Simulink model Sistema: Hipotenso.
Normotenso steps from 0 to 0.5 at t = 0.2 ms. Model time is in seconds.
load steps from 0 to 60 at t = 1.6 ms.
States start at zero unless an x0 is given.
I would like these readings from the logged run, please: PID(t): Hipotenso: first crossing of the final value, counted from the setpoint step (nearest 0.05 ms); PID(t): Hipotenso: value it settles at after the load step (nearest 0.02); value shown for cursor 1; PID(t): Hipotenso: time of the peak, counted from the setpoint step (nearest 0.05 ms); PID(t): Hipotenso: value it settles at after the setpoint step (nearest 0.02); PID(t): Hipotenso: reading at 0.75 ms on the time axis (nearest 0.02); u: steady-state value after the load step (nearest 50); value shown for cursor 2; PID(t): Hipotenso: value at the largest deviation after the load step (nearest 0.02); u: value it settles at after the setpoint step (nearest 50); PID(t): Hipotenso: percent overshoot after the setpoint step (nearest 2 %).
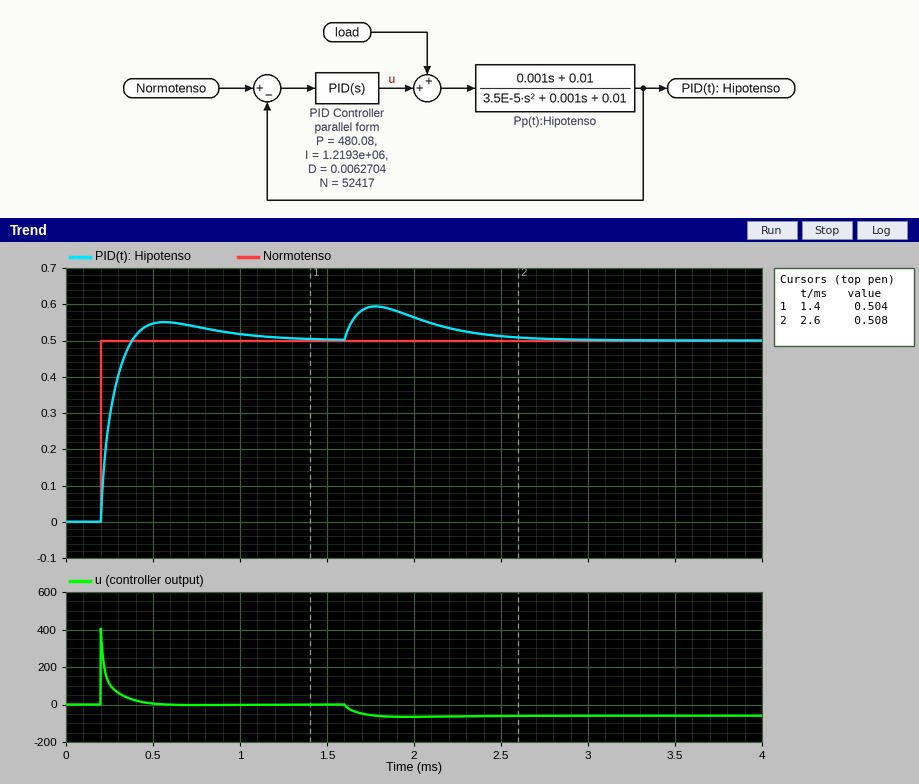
0.20 ms
0.50
0.504
0.35 ms
0.50
0.54
-50
0.508
0.60
0
10 %
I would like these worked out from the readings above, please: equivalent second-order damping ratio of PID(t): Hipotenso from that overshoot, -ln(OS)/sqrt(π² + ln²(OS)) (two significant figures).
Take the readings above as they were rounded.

0.59
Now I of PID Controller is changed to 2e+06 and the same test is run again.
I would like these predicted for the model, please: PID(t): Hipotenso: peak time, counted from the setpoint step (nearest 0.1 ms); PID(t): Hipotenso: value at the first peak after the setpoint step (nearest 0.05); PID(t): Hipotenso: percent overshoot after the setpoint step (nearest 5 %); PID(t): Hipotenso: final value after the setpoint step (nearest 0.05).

0.3 ms
0.55
15 %
0.50
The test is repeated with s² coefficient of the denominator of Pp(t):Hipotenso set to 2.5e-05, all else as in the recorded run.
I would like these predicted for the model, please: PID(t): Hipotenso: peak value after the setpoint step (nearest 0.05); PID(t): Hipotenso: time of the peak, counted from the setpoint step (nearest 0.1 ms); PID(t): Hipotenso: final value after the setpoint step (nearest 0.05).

0.55
0.3 ms
0.50
